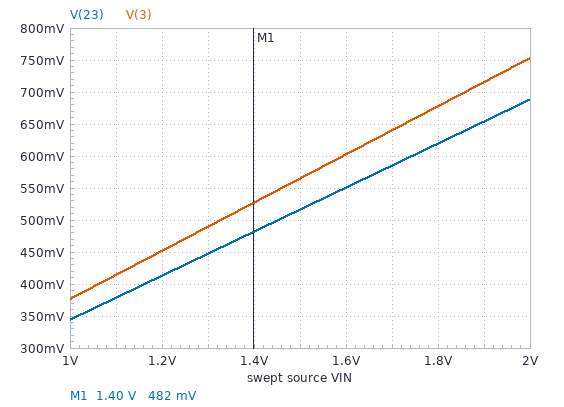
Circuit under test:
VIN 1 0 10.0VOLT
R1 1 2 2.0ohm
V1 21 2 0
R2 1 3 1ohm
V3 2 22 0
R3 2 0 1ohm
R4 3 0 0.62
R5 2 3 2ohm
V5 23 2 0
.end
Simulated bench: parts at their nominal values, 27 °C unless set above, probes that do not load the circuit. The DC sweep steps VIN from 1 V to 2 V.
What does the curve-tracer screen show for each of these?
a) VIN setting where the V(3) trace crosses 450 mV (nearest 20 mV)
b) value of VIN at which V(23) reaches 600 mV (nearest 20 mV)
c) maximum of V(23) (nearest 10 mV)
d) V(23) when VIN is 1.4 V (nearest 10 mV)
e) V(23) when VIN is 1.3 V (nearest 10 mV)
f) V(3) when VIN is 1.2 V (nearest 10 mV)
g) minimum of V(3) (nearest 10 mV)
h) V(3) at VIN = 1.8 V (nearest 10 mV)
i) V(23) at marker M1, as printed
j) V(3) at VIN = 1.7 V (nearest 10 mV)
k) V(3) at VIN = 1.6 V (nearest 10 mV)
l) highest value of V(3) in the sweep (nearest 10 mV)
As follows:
1.20 V
1.74 V
690 mV
480 mV
450 mV
450 mV
380 mV
680 mV
482 mV
640 mV
600 mV
750 mV
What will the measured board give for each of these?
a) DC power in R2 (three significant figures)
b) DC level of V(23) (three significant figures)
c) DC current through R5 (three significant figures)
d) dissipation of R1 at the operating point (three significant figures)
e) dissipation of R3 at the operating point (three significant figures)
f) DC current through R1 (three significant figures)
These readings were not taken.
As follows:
38.9 W
3.44 V
162 mA
21.5 W
11.8 W
3.28 A
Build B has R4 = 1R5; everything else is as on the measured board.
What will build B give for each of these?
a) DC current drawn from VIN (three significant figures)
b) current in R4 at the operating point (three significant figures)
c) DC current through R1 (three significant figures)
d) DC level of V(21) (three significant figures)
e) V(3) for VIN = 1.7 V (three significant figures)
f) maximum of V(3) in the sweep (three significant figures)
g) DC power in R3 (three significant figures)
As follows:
7.55 A
3.67 A
3.06 A
3.88 V
937 mV
1.10 V
15.0 W
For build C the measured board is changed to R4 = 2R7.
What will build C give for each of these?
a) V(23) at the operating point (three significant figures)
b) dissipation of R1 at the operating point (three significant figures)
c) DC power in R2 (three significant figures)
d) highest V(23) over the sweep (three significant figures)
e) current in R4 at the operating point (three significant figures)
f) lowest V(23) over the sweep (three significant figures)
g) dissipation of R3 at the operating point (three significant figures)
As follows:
4.11 V
17.3 W
12.6 W
822 mV
2.39 A
411 mV
16.9 W
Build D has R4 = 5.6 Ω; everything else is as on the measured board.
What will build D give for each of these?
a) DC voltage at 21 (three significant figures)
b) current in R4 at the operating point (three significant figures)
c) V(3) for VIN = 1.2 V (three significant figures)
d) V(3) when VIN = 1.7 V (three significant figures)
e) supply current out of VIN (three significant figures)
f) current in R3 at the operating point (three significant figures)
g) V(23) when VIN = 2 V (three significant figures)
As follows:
4.31 V
1.29 A
869 mV
1.23 V
5.60 A
4.31 A
862 mV
